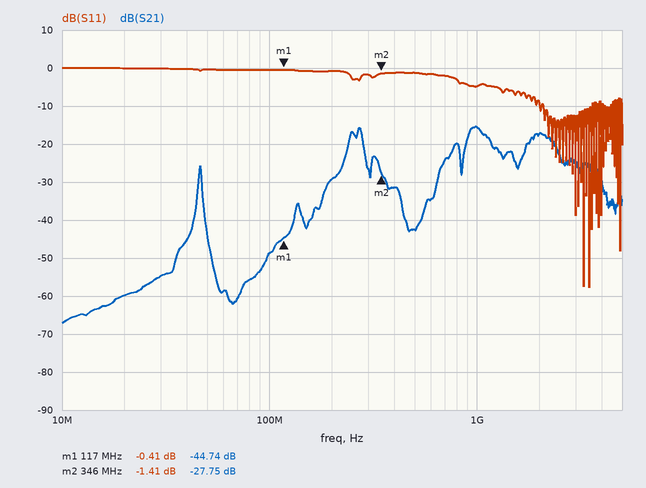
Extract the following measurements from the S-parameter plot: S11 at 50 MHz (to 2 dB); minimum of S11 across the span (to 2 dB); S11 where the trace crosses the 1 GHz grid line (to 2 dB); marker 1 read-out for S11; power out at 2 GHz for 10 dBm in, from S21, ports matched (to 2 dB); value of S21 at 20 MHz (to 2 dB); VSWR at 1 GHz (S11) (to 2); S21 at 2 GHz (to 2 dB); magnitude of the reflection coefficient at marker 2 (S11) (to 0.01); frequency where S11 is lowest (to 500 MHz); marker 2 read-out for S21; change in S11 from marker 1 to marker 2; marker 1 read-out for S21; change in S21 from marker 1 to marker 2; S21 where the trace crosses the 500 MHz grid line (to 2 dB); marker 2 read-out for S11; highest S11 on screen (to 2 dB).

0 dB
-58 dB
-4 dB
-0.41 dB
-8 dBm
-60 dB
4
-18 dB
0.85
3.5 GHz
-27.75 dB
-1.00 dB
-44.74 dB
16.99 dB
-42 dB
-1.41 dB
0 dB
